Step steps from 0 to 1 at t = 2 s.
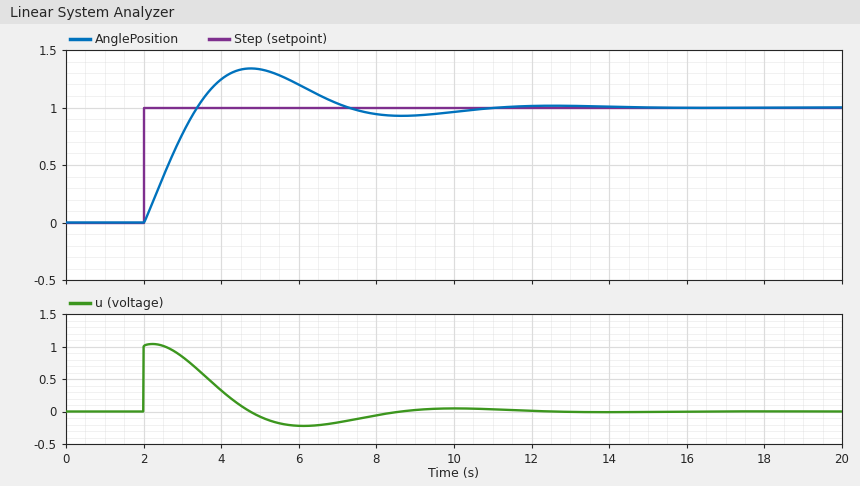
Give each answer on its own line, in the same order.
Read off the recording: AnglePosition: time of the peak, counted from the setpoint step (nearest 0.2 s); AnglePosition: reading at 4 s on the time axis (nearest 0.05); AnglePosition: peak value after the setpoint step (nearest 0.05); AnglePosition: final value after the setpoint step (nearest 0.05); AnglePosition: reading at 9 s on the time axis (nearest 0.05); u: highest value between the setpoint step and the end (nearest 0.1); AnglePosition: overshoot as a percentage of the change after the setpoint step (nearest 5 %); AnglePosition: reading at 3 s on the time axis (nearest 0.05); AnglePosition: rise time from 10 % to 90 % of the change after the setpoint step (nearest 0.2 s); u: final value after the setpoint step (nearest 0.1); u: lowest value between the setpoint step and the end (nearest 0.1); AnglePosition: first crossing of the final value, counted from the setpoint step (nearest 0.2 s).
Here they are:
2.8 s
1.25
1.35
1.00
0.95
1.0
35 %
0.75
1.0 s
0.0
-0.2
1.4 s
